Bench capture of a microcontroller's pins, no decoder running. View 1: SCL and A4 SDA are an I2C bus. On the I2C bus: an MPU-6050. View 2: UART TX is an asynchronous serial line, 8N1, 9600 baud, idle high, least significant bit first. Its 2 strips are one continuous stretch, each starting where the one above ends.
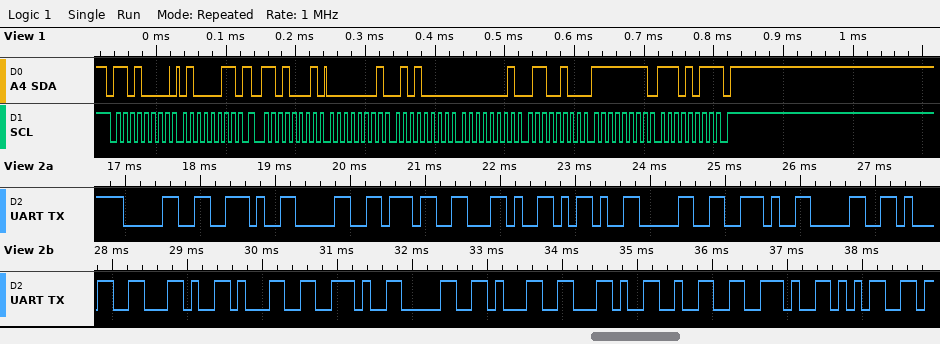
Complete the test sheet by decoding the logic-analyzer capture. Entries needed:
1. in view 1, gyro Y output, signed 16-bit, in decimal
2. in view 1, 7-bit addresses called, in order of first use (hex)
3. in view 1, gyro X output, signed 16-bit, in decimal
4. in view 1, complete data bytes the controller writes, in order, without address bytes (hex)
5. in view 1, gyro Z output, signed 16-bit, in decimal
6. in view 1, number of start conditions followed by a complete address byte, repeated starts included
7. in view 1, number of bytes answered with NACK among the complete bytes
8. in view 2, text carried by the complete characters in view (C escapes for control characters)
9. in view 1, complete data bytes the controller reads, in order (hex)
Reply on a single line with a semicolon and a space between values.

356; 0x68; 336; 43; -21; 2; 1; "0.07,-0.01,1.01,2.5"; 01 50 01 64 FF EB
